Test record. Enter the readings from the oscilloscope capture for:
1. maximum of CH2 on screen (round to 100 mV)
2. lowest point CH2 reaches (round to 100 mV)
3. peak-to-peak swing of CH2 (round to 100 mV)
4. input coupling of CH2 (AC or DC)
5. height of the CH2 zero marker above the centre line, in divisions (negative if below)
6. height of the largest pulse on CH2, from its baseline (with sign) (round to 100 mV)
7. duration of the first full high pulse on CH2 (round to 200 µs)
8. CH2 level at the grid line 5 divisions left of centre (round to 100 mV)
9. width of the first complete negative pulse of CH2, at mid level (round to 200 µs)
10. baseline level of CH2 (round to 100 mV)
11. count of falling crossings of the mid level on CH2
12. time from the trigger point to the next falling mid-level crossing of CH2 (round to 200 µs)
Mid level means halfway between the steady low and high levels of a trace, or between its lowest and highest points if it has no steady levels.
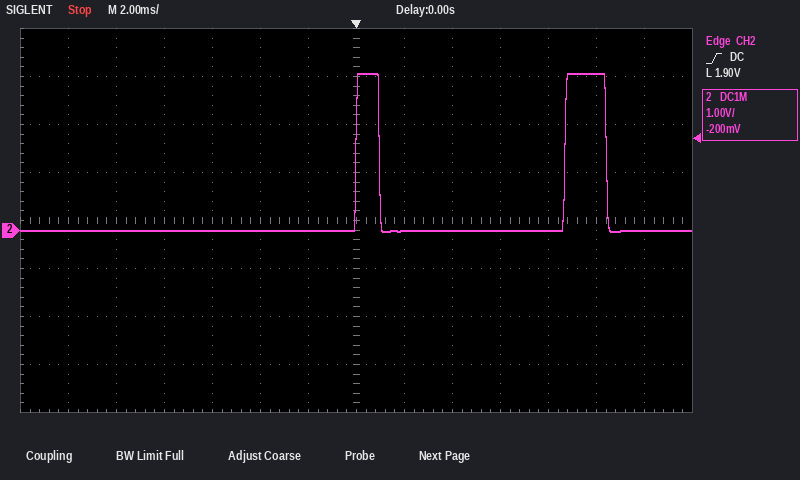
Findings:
3.3 V
0.0 V
3.3 V
DC
-0.2 div
+3.3 V
1.0 ms
0.0 V
7.8 ms
0.0 V
2
1.0 ms
